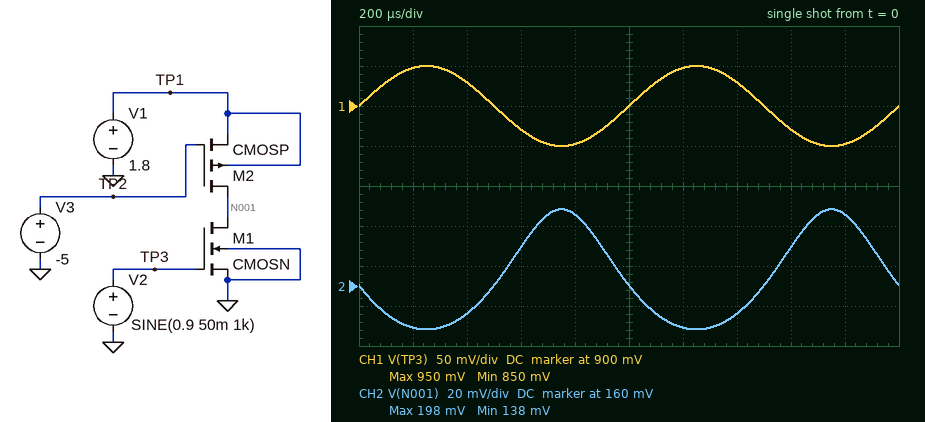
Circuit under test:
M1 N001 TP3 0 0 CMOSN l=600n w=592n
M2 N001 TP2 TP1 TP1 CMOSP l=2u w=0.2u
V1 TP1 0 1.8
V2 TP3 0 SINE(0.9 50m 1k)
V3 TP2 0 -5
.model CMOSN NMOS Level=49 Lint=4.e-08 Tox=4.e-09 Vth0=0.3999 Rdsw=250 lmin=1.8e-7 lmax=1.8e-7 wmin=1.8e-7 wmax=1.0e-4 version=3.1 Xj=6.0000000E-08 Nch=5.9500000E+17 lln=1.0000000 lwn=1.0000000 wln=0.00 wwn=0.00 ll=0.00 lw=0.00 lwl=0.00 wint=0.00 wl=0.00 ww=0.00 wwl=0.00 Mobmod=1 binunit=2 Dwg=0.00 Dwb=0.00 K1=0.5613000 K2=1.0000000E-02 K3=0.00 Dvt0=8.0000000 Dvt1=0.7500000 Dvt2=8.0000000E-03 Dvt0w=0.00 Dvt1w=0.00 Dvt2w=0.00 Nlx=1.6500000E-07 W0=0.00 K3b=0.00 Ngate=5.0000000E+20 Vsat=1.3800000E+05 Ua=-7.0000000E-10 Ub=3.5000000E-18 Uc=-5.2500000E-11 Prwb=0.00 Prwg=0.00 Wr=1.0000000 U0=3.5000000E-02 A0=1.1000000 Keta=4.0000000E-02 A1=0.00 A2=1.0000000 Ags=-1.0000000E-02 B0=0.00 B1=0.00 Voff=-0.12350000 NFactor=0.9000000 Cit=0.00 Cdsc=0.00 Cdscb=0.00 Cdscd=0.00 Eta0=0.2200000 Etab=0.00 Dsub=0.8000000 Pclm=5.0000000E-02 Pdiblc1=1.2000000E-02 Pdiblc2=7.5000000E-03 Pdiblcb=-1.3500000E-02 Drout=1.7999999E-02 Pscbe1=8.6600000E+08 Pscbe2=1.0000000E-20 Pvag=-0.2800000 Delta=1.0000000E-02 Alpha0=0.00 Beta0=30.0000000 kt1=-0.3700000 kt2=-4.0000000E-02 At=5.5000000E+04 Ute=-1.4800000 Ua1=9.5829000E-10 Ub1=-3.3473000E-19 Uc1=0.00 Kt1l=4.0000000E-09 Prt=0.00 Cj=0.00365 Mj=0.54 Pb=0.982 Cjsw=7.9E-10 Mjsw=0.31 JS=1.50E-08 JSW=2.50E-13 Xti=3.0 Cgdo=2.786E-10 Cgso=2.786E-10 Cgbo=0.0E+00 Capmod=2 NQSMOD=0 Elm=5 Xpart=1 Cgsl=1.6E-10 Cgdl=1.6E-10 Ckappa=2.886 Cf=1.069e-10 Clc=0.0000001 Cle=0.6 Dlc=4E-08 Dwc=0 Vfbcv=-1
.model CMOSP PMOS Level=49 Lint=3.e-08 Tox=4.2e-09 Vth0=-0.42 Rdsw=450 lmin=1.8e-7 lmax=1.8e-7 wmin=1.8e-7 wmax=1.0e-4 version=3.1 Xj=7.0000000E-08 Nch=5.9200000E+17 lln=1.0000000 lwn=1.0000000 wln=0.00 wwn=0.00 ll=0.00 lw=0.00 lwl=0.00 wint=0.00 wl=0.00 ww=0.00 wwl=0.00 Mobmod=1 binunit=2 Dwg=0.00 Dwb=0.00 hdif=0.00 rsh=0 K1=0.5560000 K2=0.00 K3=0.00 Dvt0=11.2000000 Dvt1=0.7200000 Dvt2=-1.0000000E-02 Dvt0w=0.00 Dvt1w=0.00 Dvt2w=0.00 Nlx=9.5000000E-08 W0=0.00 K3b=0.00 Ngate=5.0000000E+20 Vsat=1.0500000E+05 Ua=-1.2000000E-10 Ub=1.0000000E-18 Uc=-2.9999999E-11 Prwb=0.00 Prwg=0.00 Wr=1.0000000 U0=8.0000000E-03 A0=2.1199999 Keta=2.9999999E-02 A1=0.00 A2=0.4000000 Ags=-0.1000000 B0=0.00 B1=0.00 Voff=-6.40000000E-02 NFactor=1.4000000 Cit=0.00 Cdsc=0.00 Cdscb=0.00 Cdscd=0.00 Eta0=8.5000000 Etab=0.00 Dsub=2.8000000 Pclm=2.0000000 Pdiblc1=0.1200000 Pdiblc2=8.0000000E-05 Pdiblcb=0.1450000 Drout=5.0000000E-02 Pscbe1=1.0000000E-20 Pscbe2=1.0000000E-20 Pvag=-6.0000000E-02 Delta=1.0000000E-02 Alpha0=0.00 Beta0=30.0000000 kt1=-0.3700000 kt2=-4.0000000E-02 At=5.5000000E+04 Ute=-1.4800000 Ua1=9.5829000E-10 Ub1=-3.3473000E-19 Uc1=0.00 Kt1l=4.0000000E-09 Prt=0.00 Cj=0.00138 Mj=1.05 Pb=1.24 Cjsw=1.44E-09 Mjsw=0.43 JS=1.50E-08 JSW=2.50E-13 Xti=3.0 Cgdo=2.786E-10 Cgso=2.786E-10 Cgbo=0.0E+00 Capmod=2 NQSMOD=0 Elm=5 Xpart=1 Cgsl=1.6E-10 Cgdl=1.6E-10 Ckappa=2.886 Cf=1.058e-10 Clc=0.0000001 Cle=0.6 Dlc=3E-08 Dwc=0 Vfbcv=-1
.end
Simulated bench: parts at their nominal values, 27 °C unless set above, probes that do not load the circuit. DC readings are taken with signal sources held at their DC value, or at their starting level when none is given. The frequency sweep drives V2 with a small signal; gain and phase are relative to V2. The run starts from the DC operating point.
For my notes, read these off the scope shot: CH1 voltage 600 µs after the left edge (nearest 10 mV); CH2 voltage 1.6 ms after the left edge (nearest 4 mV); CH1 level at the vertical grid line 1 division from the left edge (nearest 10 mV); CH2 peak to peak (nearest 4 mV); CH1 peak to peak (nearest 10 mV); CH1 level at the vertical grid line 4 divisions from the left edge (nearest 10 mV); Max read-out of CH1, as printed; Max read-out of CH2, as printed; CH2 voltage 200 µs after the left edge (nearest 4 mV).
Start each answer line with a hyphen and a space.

- 870 mV
- 180 mV
- 950 mV
- 60 mV
- 100 mV
- 850 mV
- 950 mV
- 198 mV
- 140 mV
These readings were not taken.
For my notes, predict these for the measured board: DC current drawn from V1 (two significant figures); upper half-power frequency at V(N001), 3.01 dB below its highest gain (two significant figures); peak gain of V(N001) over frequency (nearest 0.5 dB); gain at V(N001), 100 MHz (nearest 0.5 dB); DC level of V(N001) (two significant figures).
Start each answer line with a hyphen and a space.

- 14 µA
- 1.9 GHz
- -5.0 dB
- -5.0 dB
- 160 mV
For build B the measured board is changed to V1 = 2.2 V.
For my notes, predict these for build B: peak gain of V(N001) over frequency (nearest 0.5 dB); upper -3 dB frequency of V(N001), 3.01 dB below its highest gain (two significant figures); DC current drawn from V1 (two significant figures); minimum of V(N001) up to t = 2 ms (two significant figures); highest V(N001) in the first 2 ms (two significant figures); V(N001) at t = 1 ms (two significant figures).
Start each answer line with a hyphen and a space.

- -2.0 dB
- 1.7 GHz
- 16 µA
- 160 mV
- 260 mV
- 190 mV
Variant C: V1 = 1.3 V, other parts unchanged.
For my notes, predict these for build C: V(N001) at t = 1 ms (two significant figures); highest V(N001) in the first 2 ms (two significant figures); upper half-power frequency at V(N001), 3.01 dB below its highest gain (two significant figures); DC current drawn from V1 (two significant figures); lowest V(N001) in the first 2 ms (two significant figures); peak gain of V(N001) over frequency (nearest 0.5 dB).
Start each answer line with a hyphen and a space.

- 120 mV
- 140 mV
- 3.5 GHz
- 11 µA
- 100 mV
- -9.5 dB
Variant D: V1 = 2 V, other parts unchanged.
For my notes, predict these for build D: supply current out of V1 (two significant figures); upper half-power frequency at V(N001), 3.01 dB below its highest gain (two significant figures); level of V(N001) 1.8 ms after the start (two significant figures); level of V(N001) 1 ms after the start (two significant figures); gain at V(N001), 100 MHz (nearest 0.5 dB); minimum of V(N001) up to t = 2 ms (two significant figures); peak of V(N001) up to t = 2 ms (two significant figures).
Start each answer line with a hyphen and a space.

- 15 µA
- 1.8 GHz
- 220 mV
- 180 mV
- -3.5 dB
- 150 mV
- 230 mV
